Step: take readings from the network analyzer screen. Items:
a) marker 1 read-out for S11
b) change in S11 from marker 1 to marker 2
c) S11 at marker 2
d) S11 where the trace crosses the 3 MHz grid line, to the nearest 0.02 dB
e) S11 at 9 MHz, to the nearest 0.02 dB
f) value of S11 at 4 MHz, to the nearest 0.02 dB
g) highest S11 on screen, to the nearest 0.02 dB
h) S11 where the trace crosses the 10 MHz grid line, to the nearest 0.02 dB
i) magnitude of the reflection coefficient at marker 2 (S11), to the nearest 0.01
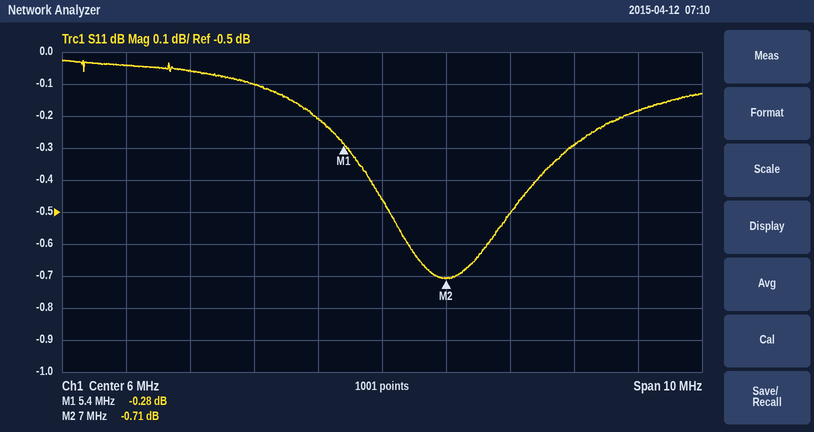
-0.28 dB
-0.43 dB
-0.71 dB
-0.06 dB
-0.30 dB
-0.10 dB
-0.02 dB
-0.18 dB
0.92
